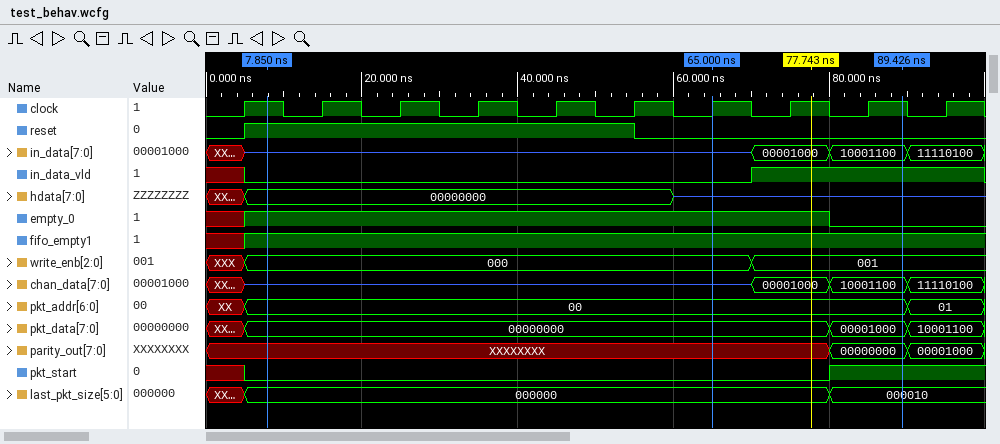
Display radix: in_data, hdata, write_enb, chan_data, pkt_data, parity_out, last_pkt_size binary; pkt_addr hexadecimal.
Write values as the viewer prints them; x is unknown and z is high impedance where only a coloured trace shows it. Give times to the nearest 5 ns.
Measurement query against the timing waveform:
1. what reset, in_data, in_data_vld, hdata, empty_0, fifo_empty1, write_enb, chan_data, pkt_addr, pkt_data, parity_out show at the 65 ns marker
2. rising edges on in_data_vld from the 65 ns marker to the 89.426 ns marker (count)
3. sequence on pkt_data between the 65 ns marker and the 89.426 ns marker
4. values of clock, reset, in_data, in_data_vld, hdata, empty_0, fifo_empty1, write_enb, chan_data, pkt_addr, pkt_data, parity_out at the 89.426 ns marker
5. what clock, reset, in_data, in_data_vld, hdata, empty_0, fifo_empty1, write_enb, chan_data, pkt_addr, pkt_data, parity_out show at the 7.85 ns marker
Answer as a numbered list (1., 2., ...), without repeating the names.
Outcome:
1. reset=0, in_data=z, in_data_vld=0, hdata=z, empty_0=1, fifo_empty1=1, write_enb=000, chan_data=z, pkt_addr=00, pkt_data=00000000, parity_out=XXXXXXXX
2. 1
3. 00000000, 00001000
4. clock=1, reset=0, in_data=10001100, in_data_vld=1, hdata=z, empty_0=0, fifo_empty1=1, write_enb=001, chan_data=10001100, pkt_addr=00, pkt_data=00001000, parity_out=00000000
5. clock=1, reset=1, in_data=z, in_data_vld=0, hdata=00000000, empty_0=1, fifo_empty1=1, write_enb=000, chan_data=z, pkt_addr=00, pkt_data=00000000, parity_out=XXXXXXXX
